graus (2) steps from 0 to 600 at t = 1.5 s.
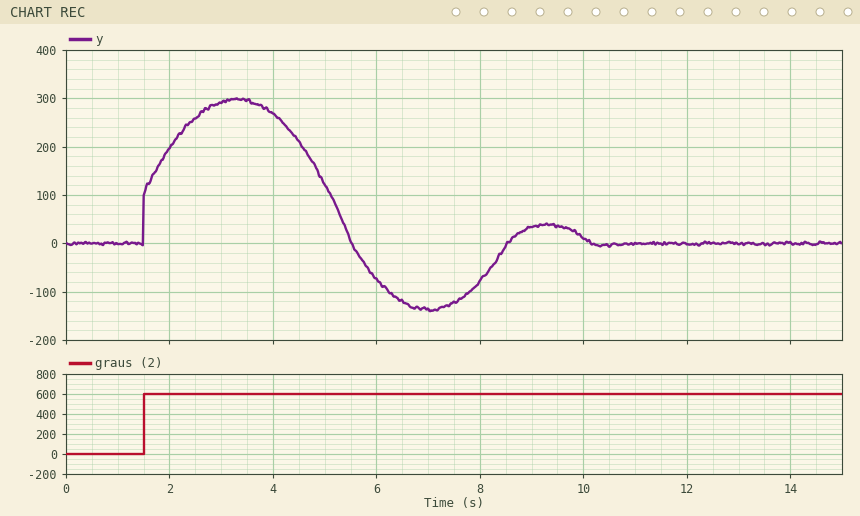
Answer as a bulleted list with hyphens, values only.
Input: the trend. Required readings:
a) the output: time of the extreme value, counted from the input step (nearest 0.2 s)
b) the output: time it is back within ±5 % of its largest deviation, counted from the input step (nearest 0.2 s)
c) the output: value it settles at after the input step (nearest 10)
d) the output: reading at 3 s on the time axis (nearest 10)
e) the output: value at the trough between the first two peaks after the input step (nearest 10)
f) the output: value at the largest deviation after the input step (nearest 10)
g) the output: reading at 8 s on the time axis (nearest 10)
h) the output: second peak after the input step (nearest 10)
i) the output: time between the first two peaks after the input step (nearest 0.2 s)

- 1.8 s
- 8.4 s
- 0
- 290
- -140
- 300
- -80
- 40
- 6.0 s
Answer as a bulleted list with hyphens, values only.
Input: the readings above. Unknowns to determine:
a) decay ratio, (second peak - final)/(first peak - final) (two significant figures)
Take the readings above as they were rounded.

- 0.13
